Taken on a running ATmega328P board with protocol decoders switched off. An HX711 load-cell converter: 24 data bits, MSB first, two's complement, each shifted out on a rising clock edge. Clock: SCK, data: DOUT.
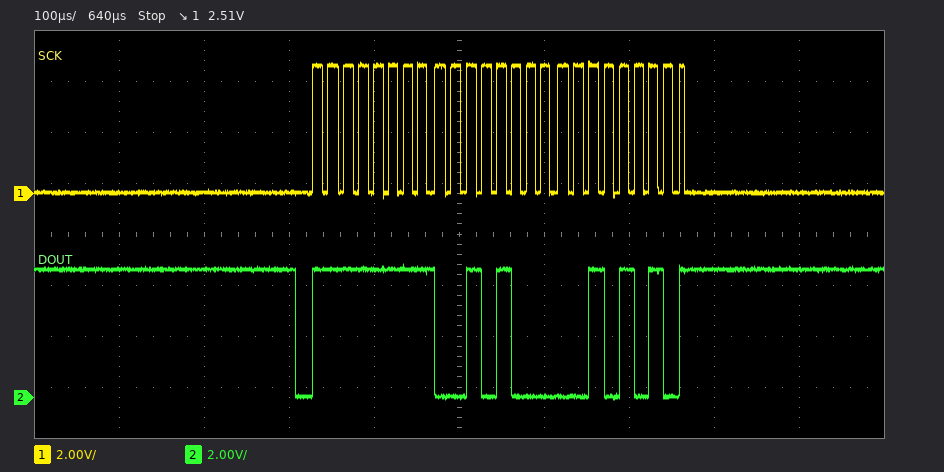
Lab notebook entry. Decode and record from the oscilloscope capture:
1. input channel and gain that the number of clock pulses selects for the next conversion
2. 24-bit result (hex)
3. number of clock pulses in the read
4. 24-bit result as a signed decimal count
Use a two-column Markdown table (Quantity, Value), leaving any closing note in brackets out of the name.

| Quantity | Value |
|---|---|
| input channel and gain that the number of clock pulses selects for the next conversion | channel A, gain 128 |
| 24-bit result | 0xFF282A |
| number of clock pulses in the read | 25 |
| 24-bit result as a signed decimal count | -55254 |
